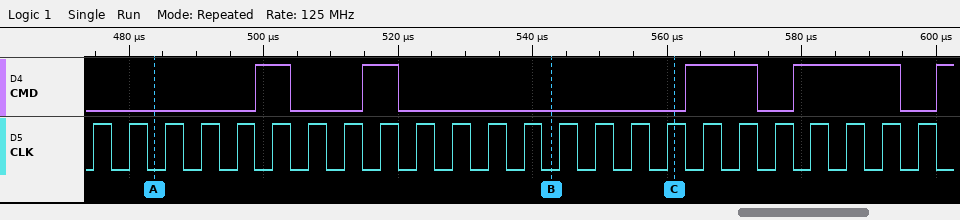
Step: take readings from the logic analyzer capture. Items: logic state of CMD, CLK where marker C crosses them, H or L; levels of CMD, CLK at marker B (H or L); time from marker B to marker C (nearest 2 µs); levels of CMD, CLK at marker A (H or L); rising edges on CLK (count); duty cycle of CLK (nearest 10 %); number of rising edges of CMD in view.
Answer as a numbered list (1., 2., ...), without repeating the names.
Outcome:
1. CMD=L, CLK=H
2. CMD=L, CLK=L
3. 18 µs
4. CMD=L, CLK=L
5. 24
6. 50 %
7. 5
